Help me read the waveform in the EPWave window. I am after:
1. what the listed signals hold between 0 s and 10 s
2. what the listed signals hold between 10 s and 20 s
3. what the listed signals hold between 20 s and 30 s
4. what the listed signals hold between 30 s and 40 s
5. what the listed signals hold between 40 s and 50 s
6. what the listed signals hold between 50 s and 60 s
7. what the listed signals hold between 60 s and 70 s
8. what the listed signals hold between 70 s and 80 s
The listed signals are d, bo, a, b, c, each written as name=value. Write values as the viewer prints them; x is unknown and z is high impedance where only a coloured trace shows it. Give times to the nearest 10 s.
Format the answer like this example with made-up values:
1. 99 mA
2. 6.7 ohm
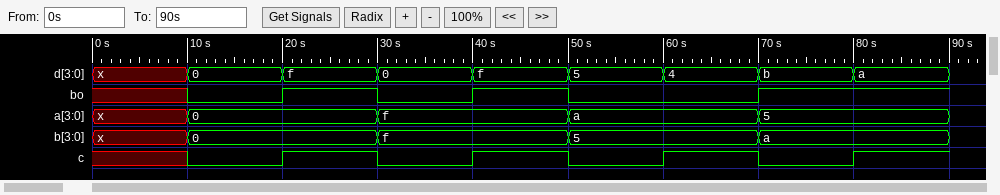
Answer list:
1. d=x, bo=x, a=x, b=x, c=x
2. d=0, bo=0, a=0, b=0, c=0
3. d=f, bo=1, a=0, b=0, c=1
4. d=0, bo=0, a=f, b=f, c=0
5. d=f, bo=1, a=f, b=f, c=1
6. d=5, bo=0, a=a, b=5, c=0
7. d=4, bo=0, a=a, b=5, c=1
8. d=b, bo=1, a=5, b=a, c=0
